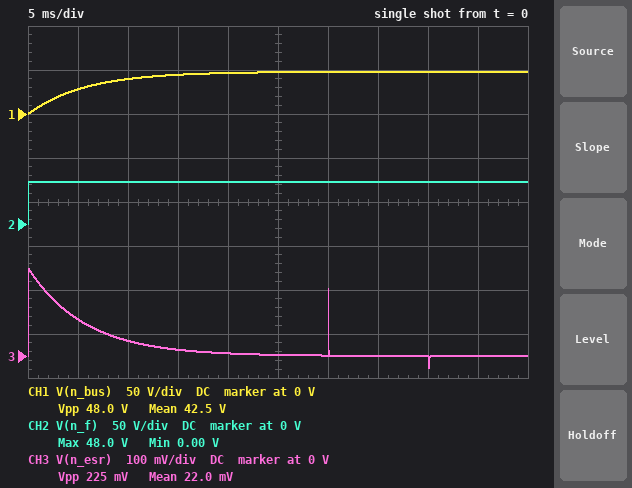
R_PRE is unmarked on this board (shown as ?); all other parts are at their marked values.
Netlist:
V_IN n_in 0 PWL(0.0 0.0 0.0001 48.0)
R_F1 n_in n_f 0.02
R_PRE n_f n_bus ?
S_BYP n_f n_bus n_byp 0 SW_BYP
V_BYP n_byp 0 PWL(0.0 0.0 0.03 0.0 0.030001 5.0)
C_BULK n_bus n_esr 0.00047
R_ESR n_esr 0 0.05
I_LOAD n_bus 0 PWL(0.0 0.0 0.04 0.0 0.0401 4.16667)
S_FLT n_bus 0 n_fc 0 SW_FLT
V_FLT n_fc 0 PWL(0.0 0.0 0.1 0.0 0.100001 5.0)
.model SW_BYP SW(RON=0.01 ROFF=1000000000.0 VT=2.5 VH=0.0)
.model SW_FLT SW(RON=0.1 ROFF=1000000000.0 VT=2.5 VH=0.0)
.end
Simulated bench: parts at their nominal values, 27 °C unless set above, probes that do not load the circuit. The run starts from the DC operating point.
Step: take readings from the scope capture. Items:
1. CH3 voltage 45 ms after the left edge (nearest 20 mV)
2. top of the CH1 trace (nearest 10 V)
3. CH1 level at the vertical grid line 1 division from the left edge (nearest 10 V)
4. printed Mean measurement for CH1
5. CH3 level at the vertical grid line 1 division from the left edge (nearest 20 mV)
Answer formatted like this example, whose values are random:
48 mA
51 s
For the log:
0 V
50 V
30 V
42.5 V
80 mV
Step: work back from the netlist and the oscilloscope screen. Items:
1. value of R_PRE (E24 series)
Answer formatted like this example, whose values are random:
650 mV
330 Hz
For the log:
12 Ω
